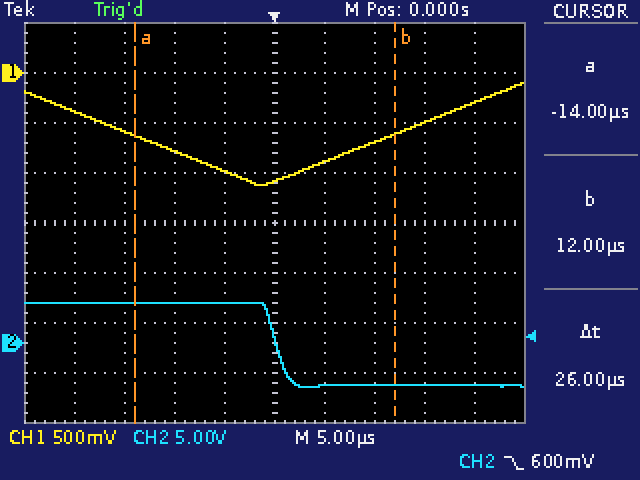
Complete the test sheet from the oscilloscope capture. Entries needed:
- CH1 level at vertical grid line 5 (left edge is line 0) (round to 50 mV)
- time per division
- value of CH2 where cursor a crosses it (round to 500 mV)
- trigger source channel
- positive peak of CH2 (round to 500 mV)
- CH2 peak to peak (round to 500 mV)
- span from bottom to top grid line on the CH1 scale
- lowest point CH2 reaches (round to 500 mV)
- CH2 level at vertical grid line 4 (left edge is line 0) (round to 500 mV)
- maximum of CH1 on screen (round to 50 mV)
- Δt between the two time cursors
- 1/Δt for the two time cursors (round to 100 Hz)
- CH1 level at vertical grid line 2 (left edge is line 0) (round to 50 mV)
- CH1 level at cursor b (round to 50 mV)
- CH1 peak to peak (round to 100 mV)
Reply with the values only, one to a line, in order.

-1.10 V
5 µs
4.0 V
CH2
4.0 V
8.5 V
4 V
-4.5 V
4.0 V
-100 mV
26 µs
38.5 kHz
-600 mV
-600 mV
1.00 V
